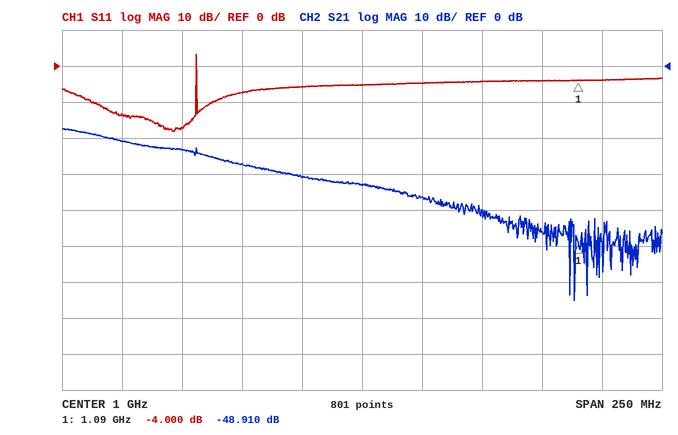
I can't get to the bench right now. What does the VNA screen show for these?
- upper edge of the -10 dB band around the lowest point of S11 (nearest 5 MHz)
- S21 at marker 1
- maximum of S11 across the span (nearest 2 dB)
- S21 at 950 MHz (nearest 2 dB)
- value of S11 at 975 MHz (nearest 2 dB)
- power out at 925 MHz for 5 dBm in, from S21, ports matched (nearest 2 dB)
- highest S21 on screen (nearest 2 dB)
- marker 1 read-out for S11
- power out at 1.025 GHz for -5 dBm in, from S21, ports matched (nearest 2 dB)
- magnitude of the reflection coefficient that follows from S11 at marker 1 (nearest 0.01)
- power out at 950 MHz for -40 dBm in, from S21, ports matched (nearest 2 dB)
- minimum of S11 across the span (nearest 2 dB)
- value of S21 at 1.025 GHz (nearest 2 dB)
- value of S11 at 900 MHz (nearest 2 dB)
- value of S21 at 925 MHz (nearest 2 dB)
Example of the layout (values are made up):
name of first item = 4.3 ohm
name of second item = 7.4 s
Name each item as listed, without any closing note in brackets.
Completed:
upper edge of the -10 dB band around the lowest point of S11 = 930 MHz
S21 at marker 1 = -48.910 dB
maximum of S11 across the span = 4 dB
S21 at 950 MHz = -28 dB
value of S11 at 975 MHz = -6 dB
power out at 925 MHz for 5 dBm in, from S21, ports matched = -18 dBm
highest S21 on screen = -18 dB
marker 1 read-out for S11 = -4.000 dB
power out at 1.025 GHz for -5 dBm in, from S21, ports matched = -42 dBm
magnitude of the reflection coefficient that follows from S11 at marker 1 = 0.63
power out at 950 MHz for -40 dBm in, from S21, ports matched = -68 dBm
minimum of S11 across the span = -18 dB
value of S21 at 1.025 GHz = -36 dB
value of S11 at 900 MHz = -14 dB
value of S21 at 925 MHz = -24 dB
